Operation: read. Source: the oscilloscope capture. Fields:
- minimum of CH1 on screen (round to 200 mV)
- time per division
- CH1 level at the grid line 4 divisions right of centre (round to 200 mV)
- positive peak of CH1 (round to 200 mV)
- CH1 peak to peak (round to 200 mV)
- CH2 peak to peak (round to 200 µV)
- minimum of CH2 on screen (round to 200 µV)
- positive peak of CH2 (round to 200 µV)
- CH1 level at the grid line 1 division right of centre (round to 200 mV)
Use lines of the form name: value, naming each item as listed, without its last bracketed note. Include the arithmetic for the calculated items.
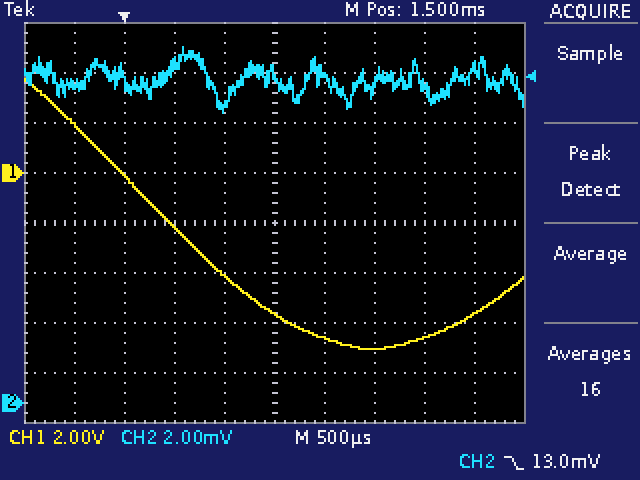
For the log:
minimum of CH1 on screen: -7.0 V
time per division: 500 µs
CH1 level at the grid line 4 divisions right of centre: -5.6 V
positive peak of CH1: 3.8 V
CH1 peak to peak: 3.8 V − (-7.0 V) = 10.8 V
CH2 peak to peak: 14.2 mV − (11.6 mV) = 2.6 mV
minimum of CH2 on screen: 11.6 mV
positive peak of CH2: 14.2 mV
CH1 level at the grid line 1 division right of centre: -6.6 V
